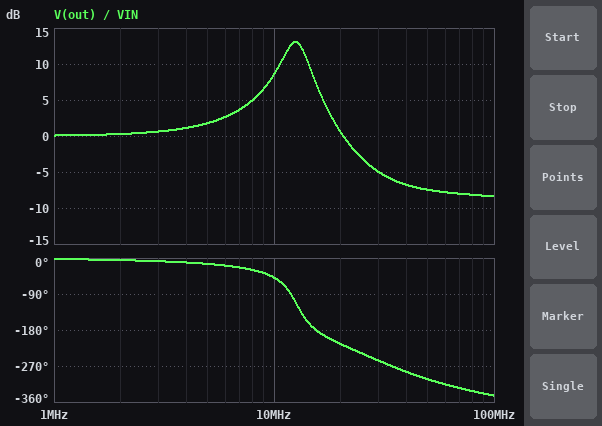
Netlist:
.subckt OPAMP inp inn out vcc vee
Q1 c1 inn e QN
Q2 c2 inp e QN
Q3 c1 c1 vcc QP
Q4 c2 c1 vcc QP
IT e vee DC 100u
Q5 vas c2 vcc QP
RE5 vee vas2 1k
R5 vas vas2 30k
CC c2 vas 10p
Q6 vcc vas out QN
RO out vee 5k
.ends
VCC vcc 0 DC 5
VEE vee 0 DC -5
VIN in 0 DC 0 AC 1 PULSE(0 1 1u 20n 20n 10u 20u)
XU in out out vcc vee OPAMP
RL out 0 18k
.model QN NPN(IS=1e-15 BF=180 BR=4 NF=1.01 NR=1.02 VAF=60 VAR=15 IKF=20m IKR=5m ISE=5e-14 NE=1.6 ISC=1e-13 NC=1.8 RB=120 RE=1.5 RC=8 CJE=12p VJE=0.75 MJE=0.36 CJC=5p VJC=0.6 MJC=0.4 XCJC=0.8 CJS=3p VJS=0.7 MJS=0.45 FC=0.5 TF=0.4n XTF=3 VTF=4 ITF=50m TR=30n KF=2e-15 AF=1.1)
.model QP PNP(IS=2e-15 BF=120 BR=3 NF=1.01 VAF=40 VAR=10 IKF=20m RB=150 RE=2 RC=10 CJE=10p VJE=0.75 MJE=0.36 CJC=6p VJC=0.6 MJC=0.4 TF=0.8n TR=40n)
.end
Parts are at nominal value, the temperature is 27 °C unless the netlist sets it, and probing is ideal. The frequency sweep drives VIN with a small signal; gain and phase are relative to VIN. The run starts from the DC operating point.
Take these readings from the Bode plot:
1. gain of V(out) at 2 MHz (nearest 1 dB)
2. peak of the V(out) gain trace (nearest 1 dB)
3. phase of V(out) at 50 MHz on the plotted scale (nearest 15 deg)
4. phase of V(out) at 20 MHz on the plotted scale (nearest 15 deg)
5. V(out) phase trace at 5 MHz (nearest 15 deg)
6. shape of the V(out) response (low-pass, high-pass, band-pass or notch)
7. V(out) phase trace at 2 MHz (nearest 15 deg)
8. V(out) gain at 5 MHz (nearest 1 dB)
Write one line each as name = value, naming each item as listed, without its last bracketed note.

gain of V(out) at 2 MHz = 0 dB
peak of the V(out) gain trace = 13 dB
phase of V(out) at 50 MHz on the plotted scale = -300 deg
phase of V(out) at 20 MHz on the plotted scale = -210 deg
V(out) phase trace at 5 MHz = -15 deg
shape of the V(out) response = band-pass
V(out) phase trace at 2 MHz = 0 deg
V(out) gain at 5 MHz = 2 dB
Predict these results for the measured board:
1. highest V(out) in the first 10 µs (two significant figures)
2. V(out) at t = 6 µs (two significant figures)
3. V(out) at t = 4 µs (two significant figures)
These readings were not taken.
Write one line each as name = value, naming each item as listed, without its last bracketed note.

highest V(out) in the first 10 µs = 1.1 V
V(out) at t = 6 µs = 1.0 V
V(out) at t = 4 µs = 1.0 V
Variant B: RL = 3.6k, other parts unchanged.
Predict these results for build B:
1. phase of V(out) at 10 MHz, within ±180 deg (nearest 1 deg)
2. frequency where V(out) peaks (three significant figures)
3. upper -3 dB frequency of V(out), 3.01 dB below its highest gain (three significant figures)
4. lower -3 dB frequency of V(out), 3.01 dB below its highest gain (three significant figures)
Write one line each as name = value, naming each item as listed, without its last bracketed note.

phase of V(out) at 10 MHz, within ±180 deg = -50 deg
frequency where V(out) peaks = 12.4 MHz
upper -3 dB frequency of V(out), 3.01 dB below its highest gain = 14.2 MHz
lower -3 dB frequency of V(out), 3.01 dB below its highest gain = 10.6 MHz
